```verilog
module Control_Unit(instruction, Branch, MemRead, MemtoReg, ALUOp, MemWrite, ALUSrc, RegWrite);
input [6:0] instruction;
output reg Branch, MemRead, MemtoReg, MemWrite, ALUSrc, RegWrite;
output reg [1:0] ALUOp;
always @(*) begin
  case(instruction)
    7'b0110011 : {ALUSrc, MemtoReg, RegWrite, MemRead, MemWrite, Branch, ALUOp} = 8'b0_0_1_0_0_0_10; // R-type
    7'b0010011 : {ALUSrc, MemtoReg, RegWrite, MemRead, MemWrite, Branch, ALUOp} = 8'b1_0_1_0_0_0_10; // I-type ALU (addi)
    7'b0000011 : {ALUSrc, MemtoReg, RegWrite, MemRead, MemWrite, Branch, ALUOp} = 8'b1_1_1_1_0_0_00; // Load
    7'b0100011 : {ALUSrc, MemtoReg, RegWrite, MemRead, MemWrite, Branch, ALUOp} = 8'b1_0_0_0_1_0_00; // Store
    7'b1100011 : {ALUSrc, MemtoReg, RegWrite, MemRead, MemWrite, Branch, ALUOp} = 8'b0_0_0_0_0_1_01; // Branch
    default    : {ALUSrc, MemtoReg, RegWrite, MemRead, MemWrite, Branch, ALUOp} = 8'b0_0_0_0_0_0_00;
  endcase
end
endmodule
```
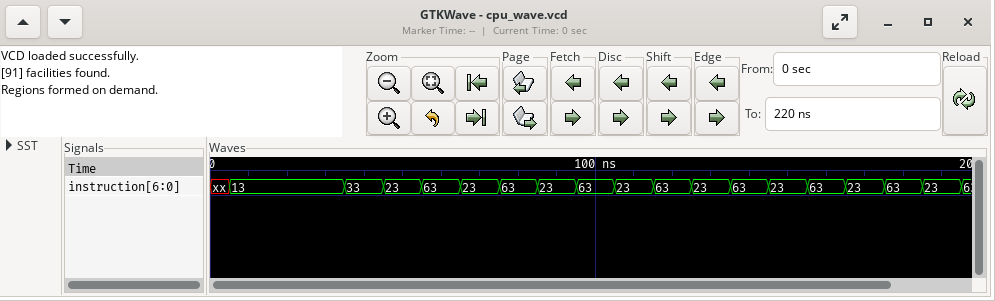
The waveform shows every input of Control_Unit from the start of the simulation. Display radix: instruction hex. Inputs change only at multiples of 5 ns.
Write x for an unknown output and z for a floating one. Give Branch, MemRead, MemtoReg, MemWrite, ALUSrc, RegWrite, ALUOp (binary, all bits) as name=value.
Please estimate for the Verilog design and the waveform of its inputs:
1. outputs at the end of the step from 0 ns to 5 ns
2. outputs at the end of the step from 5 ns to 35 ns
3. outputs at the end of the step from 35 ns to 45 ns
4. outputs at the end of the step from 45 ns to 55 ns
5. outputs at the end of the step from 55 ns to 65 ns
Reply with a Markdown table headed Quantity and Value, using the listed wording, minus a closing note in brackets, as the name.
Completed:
| Quantity | Value |
|---|---|
| outputs at the end of the step from 0 ns to 5 ns | Branch=x, MemRead=x, MemtoReg=x, MemWrite=x, ALUSrc=x, RegWrite=x, ALUOp=x |
| outputs at the end of the step from 5 ns to 35 ns | Branch=0, MemRead=0, MemtoReg=0, MemWrite=0, ALUSrc=1, RegWrite=1, ALUOp=10 |
| outputs at the end of the step from 35 ns to 45 ns | Branch=0, MemRead=0, MemtoReg=0, MemWrite=0, ALUSrc=0, RegWrite=1, ALUOp=10 |
| outputs at the end of the step from 45 ns to 55 ns | Branch=0, MemRead=0, MemtoReg=0, MemWrite=1, ALUSrc=1, RegWrite=0, ALUOp=00 |
| outputs at the end of the step from 55 ns to 65 ns | Branch=1, MemRead=0, MemtoReg=0, MemWrite=0, ALUSrc=0, RegWrite=0, ALUOp=01 |
